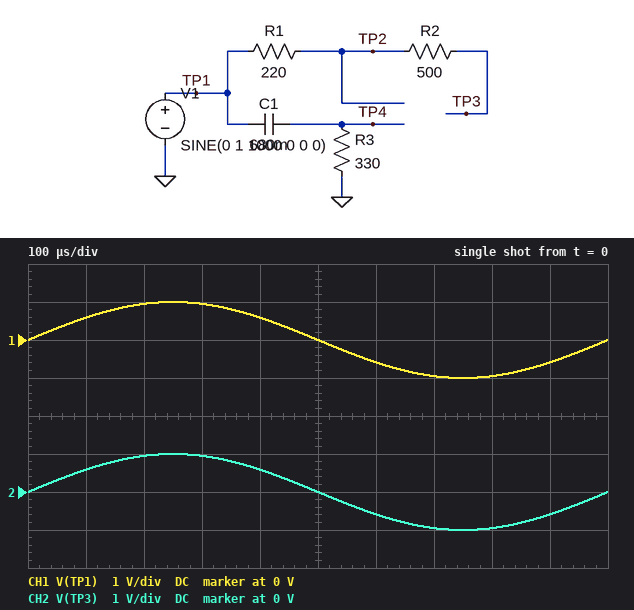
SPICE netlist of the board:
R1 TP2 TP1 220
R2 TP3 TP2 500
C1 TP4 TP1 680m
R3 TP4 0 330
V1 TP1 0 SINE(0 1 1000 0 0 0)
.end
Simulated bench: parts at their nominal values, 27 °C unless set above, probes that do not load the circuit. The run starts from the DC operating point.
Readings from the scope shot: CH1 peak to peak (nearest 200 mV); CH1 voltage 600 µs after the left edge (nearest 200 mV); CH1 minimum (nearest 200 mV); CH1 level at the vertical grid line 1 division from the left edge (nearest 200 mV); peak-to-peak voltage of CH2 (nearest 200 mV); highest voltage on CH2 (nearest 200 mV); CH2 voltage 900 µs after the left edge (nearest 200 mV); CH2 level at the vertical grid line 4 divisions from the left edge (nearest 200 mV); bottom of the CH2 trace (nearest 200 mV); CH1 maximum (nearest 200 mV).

2.0 V
-600 mV
-1.0 V
600 mV
2.0 V
1.0 V
-600 mV
600 mV
-1.0 V
1.0 V
